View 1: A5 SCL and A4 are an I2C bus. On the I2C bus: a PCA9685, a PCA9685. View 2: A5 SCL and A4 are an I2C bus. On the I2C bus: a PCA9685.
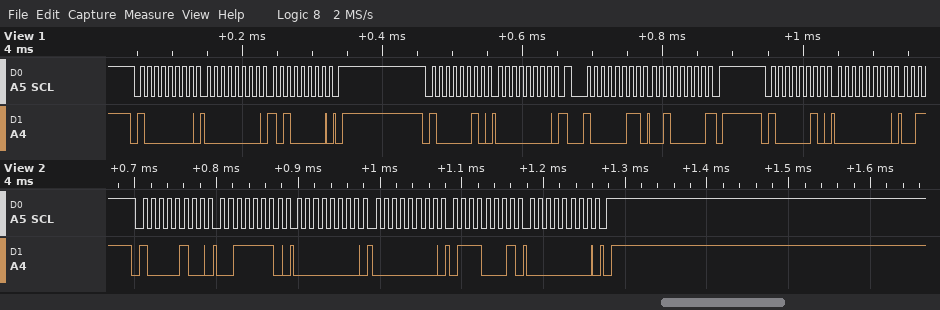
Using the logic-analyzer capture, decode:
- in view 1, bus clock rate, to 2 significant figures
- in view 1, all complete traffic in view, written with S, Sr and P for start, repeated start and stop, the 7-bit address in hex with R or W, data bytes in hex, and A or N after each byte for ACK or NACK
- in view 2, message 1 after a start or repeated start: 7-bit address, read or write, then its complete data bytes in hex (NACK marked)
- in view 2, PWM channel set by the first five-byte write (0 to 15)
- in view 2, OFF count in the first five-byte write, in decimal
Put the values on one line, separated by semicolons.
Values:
100 kHz; S 40W A 00 A A0 A P S 41W A 00 A Sr 41R A 20 N P S 41W A 00 A; 0x42 write: 3E 00 00 71 00; 14; 113
